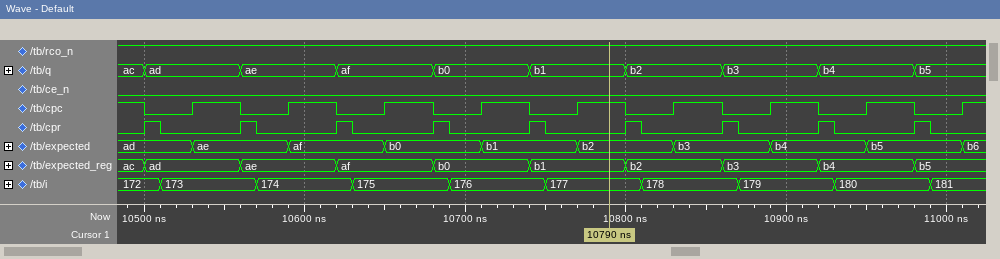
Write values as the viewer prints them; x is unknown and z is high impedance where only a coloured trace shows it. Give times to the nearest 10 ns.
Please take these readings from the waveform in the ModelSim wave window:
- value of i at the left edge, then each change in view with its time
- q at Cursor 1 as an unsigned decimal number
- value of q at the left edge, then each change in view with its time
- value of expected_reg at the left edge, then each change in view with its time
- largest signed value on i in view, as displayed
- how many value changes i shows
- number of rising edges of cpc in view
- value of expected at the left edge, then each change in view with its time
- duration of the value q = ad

172, 173 at 10510 ns, 174 at 10570 ns, 175 at 10630 ns, 176 at 10690 ns, 177 at 10750 ns, 178 at 10810 ns, 179 at 10870 ns, 180 at 10930 ns, 181 at 10990 ns
177
ac, ad at 10500 ns, ae at 10560 ns, af at 10620 ns, b0 at 10680 ns, b1 at 10740 ns, b2 at 10800 ns, b3 at 10860 ns, b4 at 10920 ns, b5 at 10980 ns
ac, ad at 10500 ns, ae at 10560 ns, af at 10620 ns, b0 at 10680 ns, b1 at 10740 ns, b2 at 10800 ns, b3 at 10860 ns, b4 at 10920 ns, b5 at 10980 ns
181
9
9
ad, ae at 10530 ns, af at 10590 ns, b0 at 10650 ns, b1 at 10710 ns, b2 at 10770 ns, b3 at 10830 ns, b4 at 10890 ns, b5 at 10950 ns, b6 at 11010 ns
60 ns
